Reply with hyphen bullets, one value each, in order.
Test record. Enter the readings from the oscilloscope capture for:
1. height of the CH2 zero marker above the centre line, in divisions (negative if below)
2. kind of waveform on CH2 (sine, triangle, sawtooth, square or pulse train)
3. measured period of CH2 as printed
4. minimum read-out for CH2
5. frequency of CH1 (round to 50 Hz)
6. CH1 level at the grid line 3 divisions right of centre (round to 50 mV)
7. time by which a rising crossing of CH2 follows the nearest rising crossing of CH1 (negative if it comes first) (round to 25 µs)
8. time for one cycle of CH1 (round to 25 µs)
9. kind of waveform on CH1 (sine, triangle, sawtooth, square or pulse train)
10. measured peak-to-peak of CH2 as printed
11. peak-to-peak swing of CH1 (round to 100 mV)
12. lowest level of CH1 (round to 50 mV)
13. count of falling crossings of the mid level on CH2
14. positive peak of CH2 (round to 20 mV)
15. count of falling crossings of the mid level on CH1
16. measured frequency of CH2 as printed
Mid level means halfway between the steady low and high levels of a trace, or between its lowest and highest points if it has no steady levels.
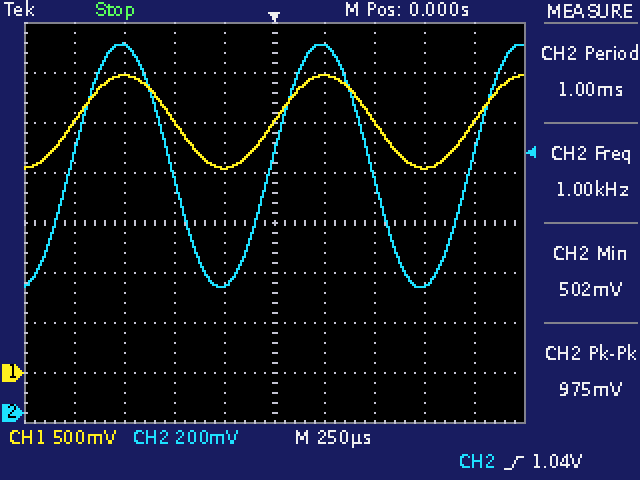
- -3.8 div
- sine
- 1.00 ms
- 502 mV
- 1.00 kHz
- 2.05 V
- -25 µs
- 1.000 ms
- sine
- 975 mV
- 900 mV
- 2.05 V
- 2
- 1.48 V
- 2
- 1.00 kHz
